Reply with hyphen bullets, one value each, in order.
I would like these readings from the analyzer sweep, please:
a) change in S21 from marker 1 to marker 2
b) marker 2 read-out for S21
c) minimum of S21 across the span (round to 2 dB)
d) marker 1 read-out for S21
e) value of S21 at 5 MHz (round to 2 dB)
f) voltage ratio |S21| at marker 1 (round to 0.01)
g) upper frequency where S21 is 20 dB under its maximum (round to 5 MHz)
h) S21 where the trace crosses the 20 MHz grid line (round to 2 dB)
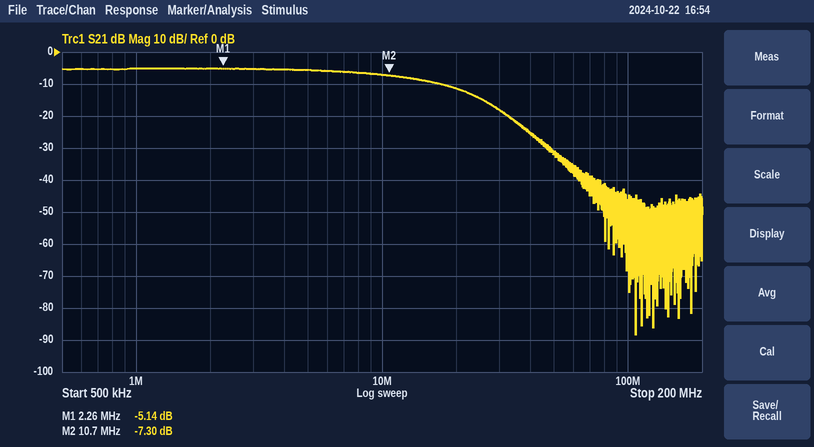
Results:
- -2.16 dB
- -7.30 dB
- -88 dB
- -5.14 dB
- -6 dB
- 0.55
- 40 MHz
- -12 dB
